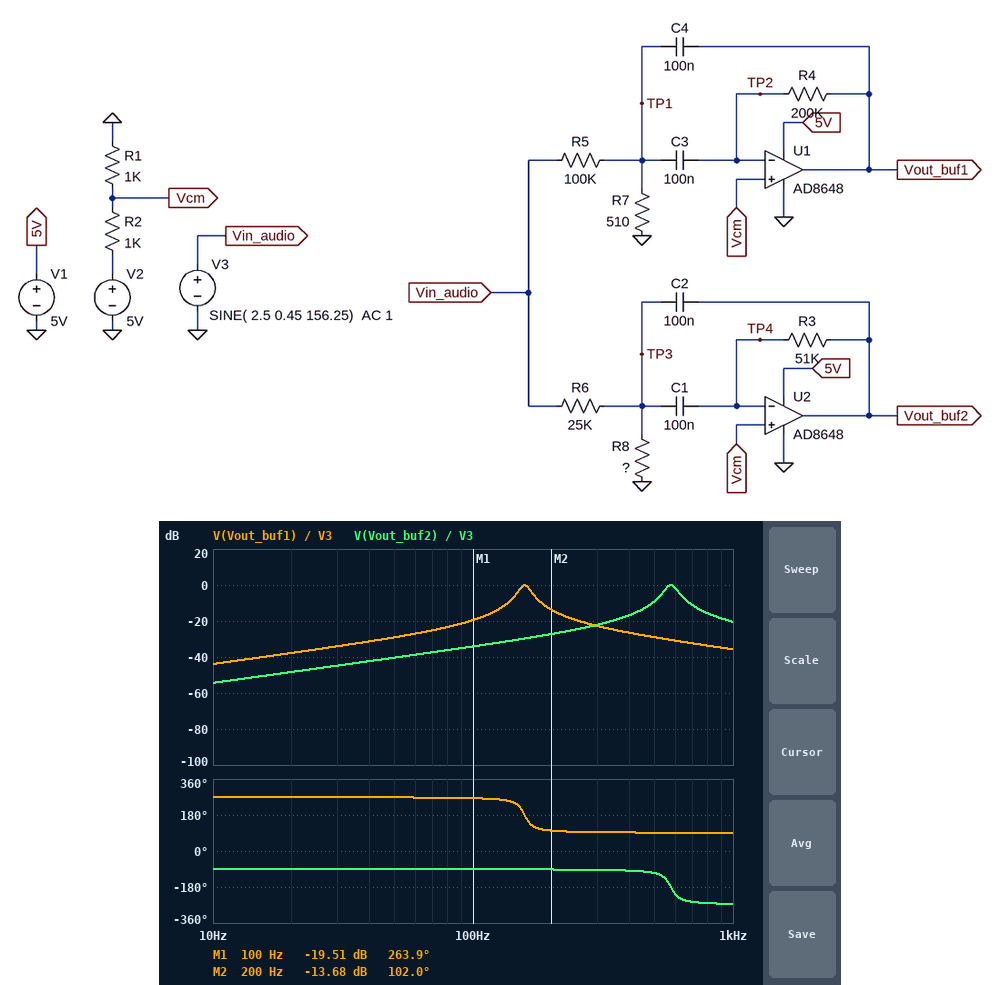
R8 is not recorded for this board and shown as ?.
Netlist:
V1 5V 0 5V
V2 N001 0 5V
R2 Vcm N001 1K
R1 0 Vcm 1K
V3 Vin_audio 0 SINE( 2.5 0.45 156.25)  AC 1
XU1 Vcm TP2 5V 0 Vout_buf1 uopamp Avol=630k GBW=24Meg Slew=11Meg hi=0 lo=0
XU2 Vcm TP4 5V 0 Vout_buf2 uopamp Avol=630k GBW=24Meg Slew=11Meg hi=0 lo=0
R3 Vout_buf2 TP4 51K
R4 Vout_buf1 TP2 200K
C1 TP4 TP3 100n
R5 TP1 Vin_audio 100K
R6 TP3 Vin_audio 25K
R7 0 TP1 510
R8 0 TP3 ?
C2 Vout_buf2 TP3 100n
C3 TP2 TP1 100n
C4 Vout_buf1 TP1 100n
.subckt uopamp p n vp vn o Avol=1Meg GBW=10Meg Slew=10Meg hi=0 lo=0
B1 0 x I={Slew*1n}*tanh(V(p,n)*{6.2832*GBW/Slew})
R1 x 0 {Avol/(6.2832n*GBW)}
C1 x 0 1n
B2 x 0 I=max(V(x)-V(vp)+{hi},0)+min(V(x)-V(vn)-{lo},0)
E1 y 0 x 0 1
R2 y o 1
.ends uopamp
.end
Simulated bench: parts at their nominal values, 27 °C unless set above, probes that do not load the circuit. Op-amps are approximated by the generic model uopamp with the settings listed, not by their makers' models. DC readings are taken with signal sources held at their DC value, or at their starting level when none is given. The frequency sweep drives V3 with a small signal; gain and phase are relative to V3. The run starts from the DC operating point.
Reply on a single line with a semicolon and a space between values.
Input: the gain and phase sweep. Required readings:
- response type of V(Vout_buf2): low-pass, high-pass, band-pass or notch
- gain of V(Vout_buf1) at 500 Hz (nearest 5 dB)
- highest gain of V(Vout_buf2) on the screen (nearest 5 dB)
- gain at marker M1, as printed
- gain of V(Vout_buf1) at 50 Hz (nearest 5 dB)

band-pass; -30 dB; 0 dB; -19.51 dB; -30 dB
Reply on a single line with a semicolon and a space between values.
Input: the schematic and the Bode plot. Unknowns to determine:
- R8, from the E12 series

150 Ω
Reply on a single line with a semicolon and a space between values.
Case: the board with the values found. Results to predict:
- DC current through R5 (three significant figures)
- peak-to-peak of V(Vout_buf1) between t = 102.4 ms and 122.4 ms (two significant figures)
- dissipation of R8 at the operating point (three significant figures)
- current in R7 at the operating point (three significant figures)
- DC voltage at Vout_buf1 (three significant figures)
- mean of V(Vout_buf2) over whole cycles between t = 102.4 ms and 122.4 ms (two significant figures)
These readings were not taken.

24.9 µA; 880 mV; 1.48 µW; 24.9 µA; 2.50 V; 2.5 V
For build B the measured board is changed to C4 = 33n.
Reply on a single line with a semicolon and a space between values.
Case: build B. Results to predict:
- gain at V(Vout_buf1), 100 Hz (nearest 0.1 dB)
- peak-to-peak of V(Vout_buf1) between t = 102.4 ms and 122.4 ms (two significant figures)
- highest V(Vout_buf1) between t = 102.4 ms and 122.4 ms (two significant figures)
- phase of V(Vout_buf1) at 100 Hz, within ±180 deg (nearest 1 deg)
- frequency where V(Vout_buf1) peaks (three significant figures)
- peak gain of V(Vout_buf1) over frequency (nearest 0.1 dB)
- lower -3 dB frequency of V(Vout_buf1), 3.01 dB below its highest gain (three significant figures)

-22.7 dB; 130 mV; 2.6 V; -93 deg; 275 Hz; 3.5 dB; 259 Hz
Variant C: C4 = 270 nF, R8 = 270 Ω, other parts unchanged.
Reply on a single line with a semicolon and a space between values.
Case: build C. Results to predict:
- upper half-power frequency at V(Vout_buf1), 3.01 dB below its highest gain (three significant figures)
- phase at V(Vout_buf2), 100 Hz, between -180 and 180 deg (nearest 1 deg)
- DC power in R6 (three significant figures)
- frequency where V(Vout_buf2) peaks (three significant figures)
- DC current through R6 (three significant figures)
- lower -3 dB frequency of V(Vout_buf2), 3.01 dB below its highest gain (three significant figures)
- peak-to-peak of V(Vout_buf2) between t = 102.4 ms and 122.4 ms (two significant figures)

102 Hz; -92 deg; 245 µW; 431 Hz; 98.9 µA; 401 Hz; 55 mV
